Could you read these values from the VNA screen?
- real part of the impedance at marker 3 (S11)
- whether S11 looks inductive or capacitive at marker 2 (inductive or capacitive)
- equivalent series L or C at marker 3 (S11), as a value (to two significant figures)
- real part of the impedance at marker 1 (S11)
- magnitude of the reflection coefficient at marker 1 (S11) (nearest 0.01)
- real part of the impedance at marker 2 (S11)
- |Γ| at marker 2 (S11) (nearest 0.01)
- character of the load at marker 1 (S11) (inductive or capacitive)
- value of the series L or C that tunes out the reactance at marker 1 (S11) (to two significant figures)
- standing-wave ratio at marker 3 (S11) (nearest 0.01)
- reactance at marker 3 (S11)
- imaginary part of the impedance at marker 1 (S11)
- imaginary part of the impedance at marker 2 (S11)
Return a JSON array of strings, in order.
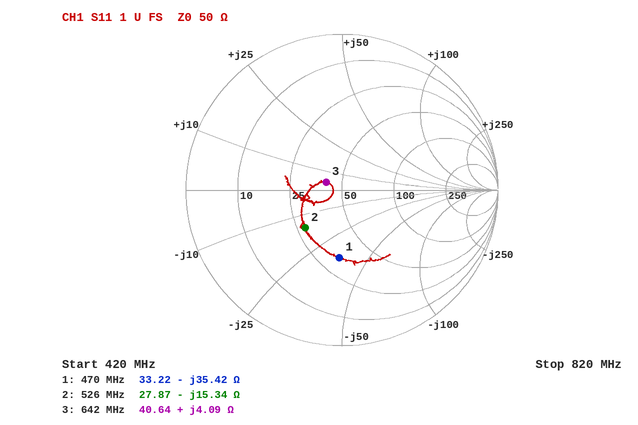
["40.64 Ω", "capacitive", "1.0 nH", "33.22 Ω", "0.43", "27.87 Ω", "0.34", "capacitive", "12 nH", "1.25", "+4.09 Ω", "-35.42 Ω", "-15.34 Ω"]
